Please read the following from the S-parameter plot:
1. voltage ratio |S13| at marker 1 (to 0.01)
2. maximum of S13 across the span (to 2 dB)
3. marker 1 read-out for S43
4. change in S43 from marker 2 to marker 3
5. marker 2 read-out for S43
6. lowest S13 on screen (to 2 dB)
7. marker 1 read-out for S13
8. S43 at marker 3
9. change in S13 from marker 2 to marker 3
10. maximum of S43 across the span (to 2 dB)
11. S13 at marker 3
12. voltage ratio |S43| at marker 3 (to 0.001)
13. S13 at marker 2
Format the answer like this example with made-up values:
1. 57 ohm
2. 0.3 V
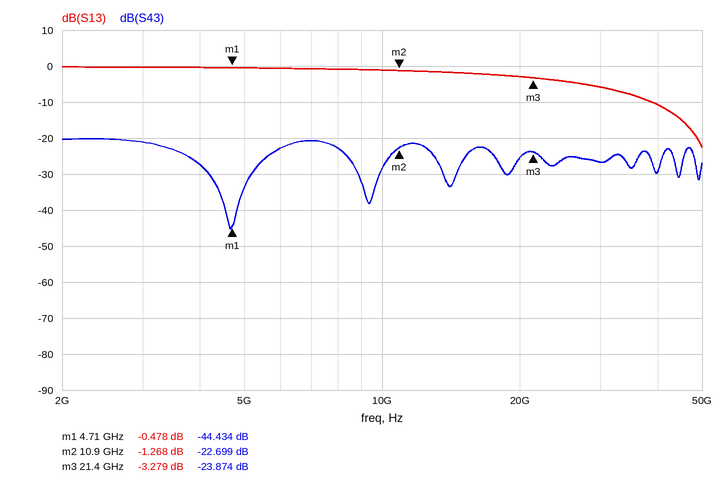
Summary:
1. 0.95
2. 0 dB
3. -44.434 dB
4. -1.175 dB
5. -22.699 dB
6. -22 dB
7. -0.478 dB
8. -23.874 dB
9. -2.011 dB
10. -20 dB
11. -3.279 dB
12. 0.064
13. -1.268 dB
